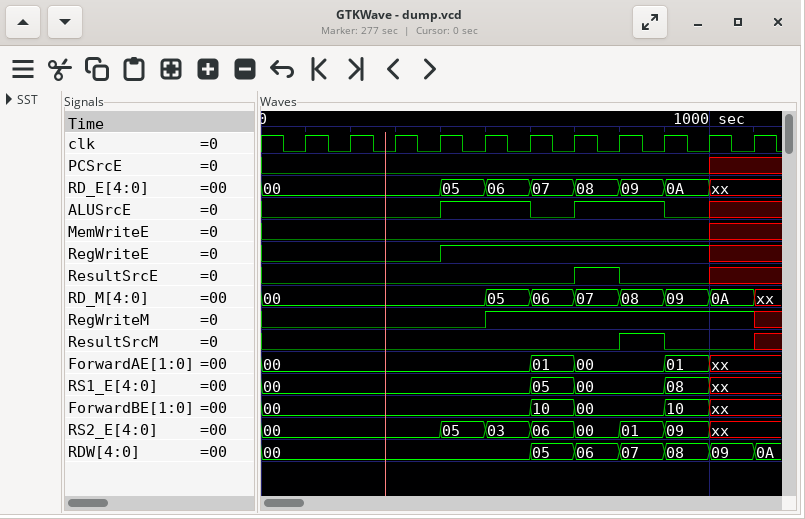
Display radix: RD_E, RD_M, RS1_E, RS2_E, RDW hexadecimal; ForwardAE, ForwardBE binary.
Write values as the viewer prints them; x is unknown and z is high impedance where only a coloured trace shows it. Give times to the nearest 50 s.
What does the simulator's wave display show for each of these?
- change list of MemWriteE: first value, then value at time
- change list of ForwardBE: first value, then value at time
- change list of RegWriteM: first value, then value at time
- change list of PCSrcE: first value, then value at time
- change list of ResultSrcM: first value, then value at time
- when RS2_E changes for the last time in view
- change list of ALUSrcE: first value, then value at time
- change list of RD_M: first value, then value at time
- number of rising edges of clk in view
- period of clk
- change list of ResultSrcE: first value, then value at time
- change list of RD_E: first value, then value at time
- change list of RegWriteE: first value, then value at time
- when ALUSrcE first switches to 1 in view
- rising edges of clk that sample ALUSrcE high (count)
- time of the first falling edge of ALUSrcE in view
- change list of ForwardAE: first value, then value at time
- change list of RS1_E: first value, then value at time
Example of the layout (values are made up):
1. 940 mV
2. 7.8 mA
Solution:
1. 0, x at 1000 s
2. 00, 10 at 600 s, 00 at 700 s, 10 at 900 s, xx at 1000 s
3. 0, 1 at 500 s, x at 1100 s
4. 0, x at 1000 s
5. 0, 1 at 800 s, 0 at 900 s, x at 1100 s
6. 1000 s
7. 0, 1 at 400 s, 0 at 600 s, 1 at 700 s, 0 at 900 s, x at 1000 s
8. 00, 05 at 500 s, 06 at 600 s, 07 at 700 s, 08 at 800 s, 09 at 900 s, 0A at 1000 s, xx at 1100 s
9. 11
10. 100 s
11. 0, 1 at 700 s, 0 at 800 s, x at 1000 s
12. 00, 05 at 400 s, 06 at 500 s, 07 at 600 s, 08 at 700 s, 09 at 800 s, 0A at 900 s, xx at 1000 s
13. 0, 1 at 400 s, x at 1000 s
14. 400 s
15. 4
16. 600 s
17. 00, 01 at 600 s, 00 at 700 s, 01 at 900 s, xx at 1000 s
18. 00, 05 at 600 s, 00 at 700 s, 08 at 900 s, xx at 1000 s
